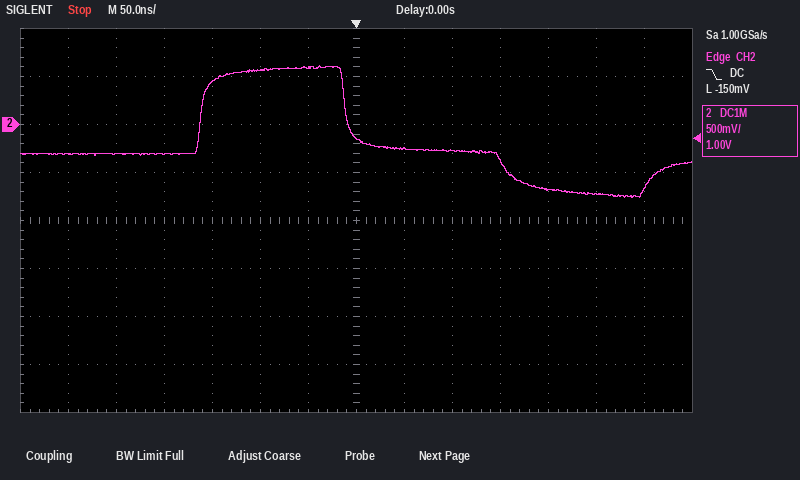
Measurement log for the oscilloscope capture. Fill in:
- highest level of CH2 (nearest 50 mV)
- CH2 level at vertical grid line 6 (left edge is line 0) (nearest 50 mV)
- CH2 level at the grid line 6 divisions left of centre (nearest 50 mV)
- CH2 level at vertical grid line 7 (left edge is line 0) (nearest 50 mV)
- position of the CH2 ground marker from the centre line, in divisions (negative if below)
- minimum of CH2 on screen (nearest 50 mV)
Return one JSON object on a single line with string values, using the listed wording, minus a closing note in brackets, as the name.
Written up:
{"highest level of CH2": "600 mV", "CH2 level at vertical grid line 6 (left edge is line 0)": "600 mV", "CH2 level at the grid line 6 divisions left of centre": "-300 mV", "CH2 level at vertical grid line 7 (left edge is line 0)": "-150 mV", "position of the CH2 ground marker from the centre line, in divisions": "+2.0 div", "minimum of CH2 on screen": "-750 mV"}
